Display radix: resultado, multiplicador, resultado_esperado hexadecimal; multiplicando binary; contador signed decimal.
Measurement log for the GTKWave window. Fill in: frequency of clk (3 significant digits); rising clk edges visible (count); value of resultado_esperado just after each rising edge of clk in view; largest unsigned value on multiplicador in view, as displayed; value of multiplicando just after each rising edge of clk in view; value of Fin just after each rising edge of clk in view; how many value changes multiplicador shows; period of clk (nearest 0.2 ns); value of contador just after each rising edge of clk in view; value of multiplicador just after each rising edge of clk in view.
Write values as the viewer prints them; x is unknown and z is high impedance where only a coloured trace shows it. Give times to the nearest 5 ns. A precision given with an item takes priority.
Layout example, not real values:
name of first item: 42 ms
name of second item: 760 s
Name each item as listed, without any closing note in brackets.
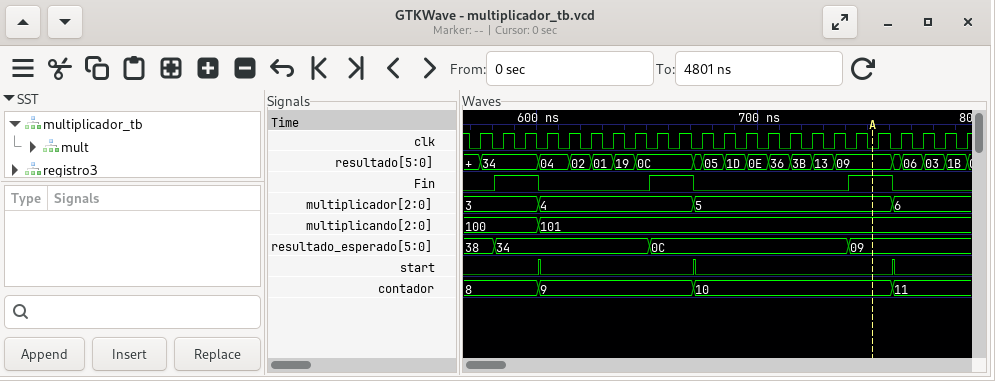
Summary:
frequency of clk: 100 MHz
rising clk edges visible: 23
value of resultado_esperado just after each rising edge of clk in view: 38, 34, 34, 34, 34, 34, 34, 34, 0C, 0C, 0C, 0C, 0C, 0C, 0C, 0C, 0C, 09, 09, 09, 09, 09, 09
largest unsigned value on multiplicador in view, as displayed: 6
value of multiplicando just after each rising edge of clk in view: 100, 100, 100, 101, 101, 101, 101, 101, 101, 101, 101, 101, 101, 101, 101, 101, 101, 101, 101, 101, 101, 101, 101
value of Fin just after each rising edge of clk in view: 0 1 1 0 0 0 0 0 1 1 0 0 0 0 0 0 0 1 1 0 0 0 0
how many value changes multiplicador shows: 3
period of clk: 10 ns
value of contador just after each rising edge of clk in view: 8, 8, 8, 9, 9, 9, 9, 9, 9, 9, 10, 10, 10, 10, 10, 10, 10, 10, 10, 11, 11, 11, 11
value of multiplicador just after each rising edge of clk in view: 3, 3, 3, 4, 4, 4, 4, 4, 4, 4, 5, 5, 5, 5, 5, 5, 5, 5, 5, 6, 6, 6, 6
